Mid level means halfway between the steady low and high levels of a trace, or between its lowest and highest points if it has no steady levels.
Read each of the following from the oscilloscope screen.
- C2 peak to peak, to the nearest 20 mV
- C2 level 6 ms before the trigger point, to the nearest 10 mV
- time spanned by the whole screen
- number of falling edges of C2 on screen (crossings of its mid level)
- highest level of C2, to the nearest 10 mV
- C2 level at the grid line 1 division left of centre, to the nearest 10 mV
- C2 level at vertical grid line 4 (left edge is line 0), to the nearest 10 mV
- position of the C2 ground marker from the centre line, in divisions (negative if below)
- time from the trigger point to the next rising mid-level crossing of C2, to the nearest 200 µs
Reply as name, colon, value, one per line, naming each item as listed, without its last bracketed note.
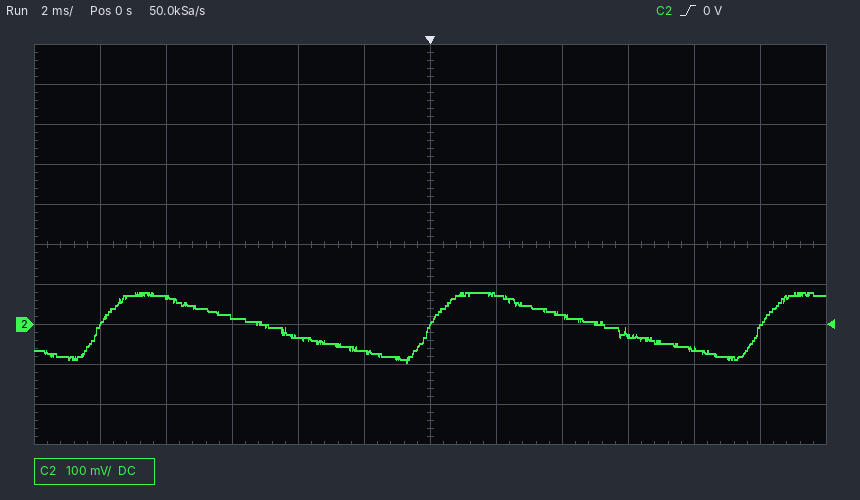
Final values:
C2 peak to peak, to the nearest 20 mV: 180 mV
C2 level 6 ms before the trigger point, to the nearest 10 mV: 20 mV
time spanned by the whole screen: 24 ms
number of falling edges of C2 on screen: 2
highest level of C2, to the nearest 10 mV: 80 mV
C2 level at the grid line 1 division left of centre, to the nearest 10 mV: -70 mV
C2 level at vertical grid line 4 (left edge is line 0), to the nearest 10 mV: -30 mV
position of the C2 ground marker from the centre line, in divisions: -2.0 div
time from the trigger point to the next rising mid-level crossing of C2, to the nearest 200 µs: 10.0 ms
